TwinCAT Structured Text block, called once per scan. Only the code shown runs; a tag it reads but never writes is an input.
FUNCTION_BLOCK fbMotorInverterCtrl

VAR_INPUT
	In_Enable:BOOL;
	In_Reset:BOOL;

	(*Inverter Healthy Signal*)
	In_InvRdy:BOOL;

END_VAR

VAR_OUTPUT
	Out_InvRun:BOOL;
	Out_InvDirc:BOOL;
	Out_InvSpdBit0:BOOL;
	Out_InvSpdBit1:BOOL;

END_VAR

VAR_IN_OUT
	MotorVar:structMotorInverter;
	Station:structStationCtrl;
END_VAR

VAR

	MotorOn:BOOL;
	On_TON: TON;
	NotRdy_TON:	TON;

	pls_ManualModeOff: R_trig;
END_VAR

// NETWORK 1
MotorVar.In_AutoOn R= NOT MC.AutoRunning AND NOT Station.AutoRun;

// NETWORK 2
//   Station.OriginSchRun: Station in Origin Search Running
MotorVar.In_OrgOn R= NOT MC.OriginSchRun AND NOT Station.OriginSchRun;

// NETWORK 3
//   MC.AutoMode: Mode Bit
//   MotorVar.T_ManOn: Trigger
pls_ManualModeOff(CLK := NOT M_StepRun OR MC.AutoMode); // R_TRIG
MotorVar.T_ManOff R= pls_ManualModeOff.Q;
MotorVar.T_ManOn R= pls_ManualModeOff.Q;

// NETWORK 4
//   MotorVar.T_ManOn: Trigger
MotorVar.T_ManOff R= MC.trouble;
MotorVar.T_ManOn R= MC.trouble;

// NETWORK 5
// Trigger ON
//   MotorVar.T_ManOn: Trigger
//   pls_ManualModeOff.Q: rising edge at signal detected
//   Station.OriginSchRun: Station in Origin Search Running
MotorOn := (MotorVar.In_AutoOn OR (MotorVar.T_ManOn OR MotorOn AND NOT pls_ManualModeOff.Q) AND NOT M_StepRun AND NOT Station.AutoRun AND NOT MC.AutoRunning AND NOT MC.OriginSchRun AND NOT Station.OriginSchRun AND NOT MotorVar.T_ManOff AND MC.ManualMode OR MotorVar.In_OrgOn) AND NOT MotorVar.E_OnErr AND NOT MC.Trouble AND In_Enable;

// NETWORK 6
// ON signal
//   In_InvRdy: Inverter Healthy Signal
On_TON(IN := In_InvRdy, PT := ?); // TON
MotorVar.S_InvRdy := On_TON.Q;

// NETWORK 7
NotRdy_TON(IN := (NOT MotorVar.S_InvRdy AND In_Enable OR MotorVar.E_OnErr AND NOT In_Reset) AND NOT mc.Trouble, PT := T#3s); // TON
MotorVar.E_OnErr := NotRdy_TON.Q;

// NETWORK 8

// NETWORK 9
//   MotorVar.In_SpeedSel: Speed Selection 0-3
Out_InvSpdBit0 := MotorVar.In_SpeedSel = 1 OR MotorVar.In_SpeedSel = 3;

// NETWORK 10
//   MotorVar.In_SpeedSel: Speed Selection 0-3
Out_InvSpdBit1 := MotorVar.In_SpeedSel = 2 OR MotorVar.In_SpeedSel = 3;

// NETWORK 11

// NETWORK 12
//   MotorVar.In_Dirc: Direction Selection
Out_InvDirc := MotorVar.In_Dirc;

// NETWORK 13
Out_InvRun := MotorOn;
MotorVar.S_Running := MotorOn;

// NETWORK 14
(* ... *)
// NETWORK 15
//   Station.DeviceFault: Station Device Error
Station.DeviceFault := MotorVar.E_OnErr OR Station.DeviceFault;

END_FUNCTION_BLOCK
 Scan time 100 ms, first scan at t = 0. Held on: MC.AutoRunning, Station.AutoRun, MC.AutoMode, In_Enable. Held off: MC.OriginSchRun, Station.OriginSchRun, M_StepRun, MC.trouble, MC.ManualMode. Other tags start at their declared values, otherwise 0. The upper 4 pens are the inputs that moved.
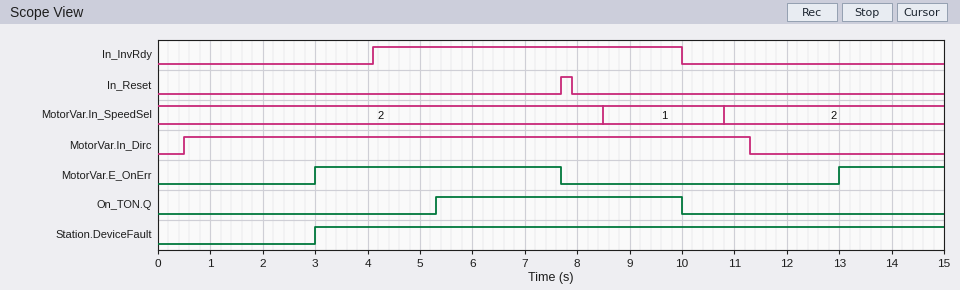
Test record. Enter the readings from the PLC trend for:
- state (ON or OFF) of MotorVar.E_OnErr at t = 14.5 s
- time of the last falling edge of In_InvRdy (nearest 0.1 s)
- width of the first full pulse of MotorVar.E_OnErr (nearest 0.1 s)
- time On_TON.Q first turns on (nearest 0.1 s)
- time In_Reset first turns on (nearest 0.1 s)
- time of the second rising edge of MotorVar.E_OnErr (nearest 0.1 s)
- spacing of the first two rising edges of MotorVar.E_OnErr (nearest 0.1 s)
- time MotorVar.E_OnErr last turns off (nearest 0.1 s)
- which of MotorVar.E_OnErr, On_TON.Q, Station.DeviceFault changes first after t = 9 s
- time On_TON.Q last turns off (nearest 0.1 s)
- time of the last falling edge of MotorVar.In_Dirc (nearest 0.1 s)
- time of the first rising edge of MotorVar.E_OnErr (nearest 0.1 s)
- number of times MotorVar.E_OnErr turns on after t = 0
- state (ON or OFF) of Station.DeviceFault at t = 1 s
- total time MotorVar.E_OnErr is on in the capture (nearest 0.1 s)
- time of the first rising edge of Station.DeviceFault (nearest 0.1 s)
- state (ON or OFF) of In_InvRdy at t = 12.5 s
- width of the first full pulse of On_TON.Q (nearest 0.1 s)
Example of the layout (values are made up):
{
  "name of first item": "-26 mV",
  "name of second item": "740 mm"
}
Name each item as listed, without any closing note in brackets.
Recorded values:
{
  "state (ON or OFF) of MotorVar.E_OnErr at t = 14.5 s": "ON",
  "time of the last falling edge of In_InvRdy": "10.0 s",
  "width of the first full pulse of MotorVar.E_OnErr": "4.7 s",
  "time On_TON.Q first turns on": "5.3 s",
  "time In_Reset first turns on": "7.7 s",
  "time of the second rising edge of MotorVar.E_OnErr": "13.0 s",
  "spacing of the first two rising edges of MotorVar.E_OnErr": "10.0 s",
  "time MotorVar.E_OnErr last turns off": "7.7 s",
  "which of MotorVar.E_OnErr, On_TON.Q, Station.DeviceFault changes first after t = 9 s": "On_TON.Q",
  "time On_TON.Q last turns off": "10.0 s",
  "time of the last falling edge of MotorVar.In_Dirc": "11.3 s",
  "time of the first rising edge of MotorVar.E_OnErr": "3.0 s",
  "number of times MotorVar.E_OnErr turns on after t = 0": "2",
  "state (ON or OFF) of Station.DeviceFault at t = 1 s": "OFF",
  "total time MotorVar.E_OnErr is on in the capture": "6.7 s",
  "time of the first rising edge of Station.DeviceFault": "3.0 s",
  "state (ON or OFF) of In_InvRdy at t = 12.5 s": "OFF",
  "width of the first full pulse of On_TON.Q": "4.7 s"
}
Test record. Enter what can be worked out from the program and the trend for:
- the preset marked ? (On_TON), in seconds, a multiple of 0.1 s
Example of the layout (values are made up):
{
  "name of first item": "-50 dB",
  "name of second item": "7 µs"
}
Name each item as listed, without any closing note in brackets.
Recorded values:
{
  "the preset marked ? (On_TON), in seconds, a multiple of 0.1 s": "1.2 s"
}
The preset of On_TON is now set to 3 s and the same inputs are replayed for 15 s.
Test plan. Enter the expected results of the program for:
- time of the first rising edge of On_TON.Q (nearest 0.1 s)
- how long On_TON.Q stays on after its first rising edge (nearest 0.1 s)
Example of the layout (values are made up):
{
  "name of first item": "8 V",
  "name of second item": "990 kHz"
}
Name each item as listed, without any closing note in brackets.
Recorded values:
{
  "time of the first rising edge of On_TON.Q": "7.1 s",
  "how long On_TON.Q stays on after its first rising edge": "2.9 s"
}
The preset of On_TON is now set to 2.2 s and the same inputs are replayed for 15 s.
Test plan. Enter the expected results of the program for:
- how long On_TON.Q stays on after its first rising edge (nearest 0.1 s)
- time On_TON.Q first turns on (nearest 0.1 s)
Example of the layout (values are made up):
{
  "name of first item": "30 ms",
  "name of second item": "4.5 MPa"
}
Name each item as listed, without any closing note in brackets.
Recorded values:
{
  "how long On_TON.Q stays on after its first rising edge": "3.7 s",
  "time On_TON.Q first turns on": "6.3 s"
}
